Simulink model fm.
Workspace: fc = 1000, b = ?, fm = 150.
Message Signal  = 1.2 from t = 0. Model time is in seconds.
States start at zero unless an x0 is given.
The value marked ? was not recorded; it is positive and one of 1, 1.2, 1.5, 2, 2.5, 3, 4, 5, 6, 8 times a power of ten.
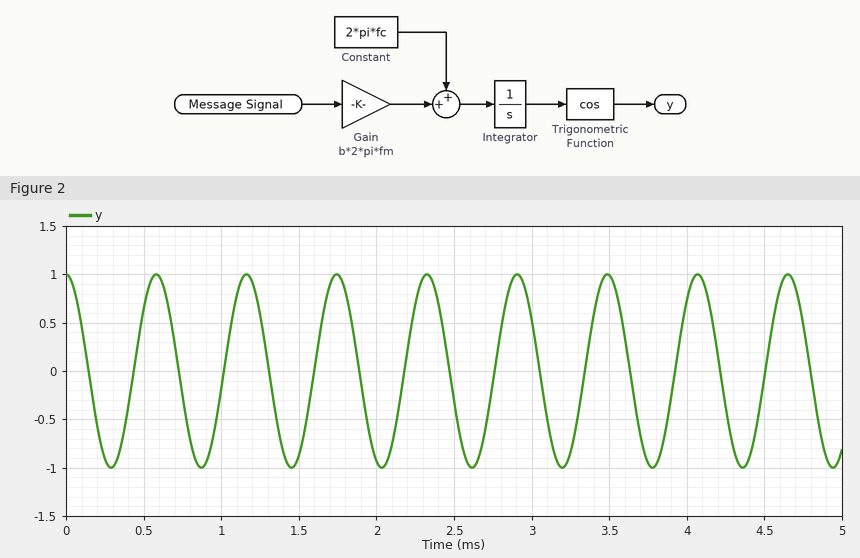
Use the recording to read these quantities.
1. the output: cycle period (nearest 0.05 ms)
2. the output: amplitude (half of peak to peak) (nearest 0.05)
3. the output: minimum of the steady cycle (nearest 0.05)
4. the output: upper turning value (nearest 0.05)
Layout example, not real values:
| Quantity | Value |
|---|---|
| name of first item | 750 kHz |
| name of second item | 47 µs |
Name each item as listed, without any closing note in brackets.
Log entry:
| Quantity | Value |
|---|---|
| the output: cycle period | 0.60 ms |
| the output: amplitude (half of peak to peak) | 1.00 |
| the output: minimum of the steady cycle | -1.00 |
| the output: upper turning value | 1.00 |
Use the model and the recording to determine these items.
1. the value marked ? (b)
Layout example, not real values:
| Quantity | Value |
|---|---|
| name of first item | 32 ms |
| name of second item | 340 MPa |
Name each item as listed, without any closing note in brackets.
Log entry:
| Quantity | Value |
|---|---|
| the value marked ? | 4 |
